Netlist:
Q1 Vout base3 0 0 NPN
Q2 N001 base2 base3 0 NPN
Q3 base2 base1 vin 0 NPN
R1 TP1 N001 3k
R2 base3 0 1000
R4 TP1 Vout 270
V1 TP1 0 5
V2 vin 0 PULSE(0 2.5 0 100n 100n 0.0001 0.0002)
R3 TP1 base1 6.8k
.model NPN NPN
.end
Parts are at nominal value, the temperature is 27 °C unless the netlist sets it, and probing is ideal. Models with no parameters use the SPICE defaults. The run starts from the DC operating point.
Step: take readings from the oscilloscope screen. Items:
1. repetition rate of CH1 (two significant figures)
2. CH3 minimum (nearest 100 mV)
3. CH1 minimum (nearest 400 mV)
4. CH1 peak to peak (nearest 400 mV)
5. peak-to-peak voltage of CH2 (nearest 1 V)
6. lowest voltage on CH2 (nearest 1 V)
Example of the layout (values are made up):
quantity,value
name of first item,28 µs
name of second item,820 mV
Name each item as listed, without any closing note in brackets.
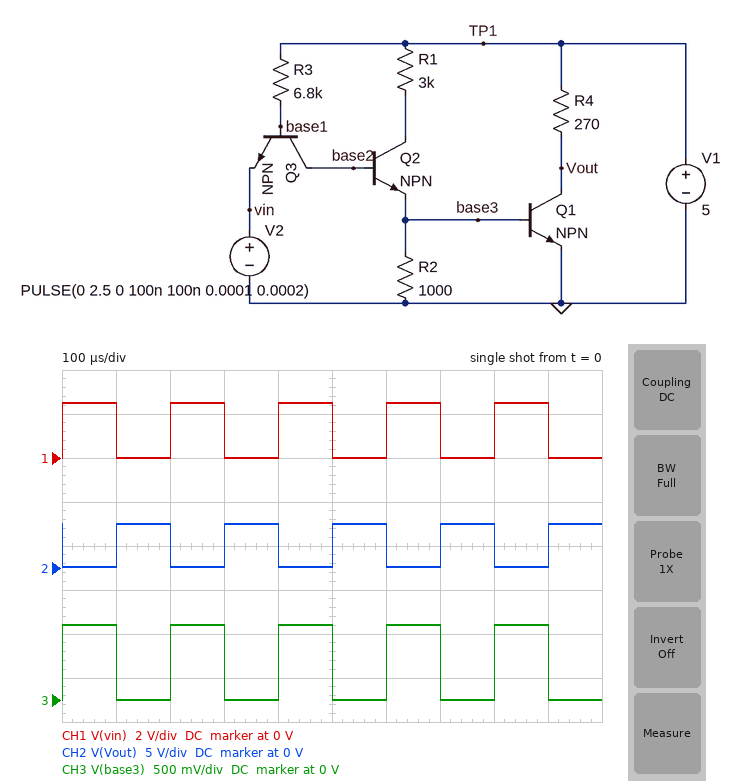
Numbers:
quantity,value
repetition rate of CH1,5.0 kHz
CH3 minimum,0 V
CH1 minimum,0 V
CH1 peak to peak,2.4 V
peak-to-peak voltage of CH2,5 V
lowest voltage on CH2,0 V
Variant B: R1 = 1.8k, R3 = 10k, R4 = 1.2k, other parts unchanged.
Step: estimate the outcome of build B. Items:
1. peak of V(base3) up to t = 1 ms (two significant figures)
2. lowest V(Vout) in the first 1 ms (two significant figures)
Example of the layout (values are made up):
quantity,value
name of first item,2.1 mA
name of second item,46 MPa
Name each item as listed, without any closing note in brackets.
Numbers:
quantity,value
peak of V(base3) up to t = 1 ms,830 mV
lowest V(Vout) in the first 1 ms,37 mV
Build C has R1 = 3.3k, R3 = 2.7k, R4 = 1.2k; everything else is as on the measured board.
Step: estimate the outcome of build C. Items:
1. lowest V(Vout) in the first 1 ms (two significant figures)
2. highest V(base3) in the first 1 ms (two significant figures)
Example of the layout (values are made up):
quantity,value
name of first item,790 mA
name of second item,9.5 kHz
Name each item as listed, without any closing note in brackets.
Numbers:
quantity,value
lowest V(Vout) in the first 1 ms,35 mV
highest V(base3) in the first 1 ms,830 mV
